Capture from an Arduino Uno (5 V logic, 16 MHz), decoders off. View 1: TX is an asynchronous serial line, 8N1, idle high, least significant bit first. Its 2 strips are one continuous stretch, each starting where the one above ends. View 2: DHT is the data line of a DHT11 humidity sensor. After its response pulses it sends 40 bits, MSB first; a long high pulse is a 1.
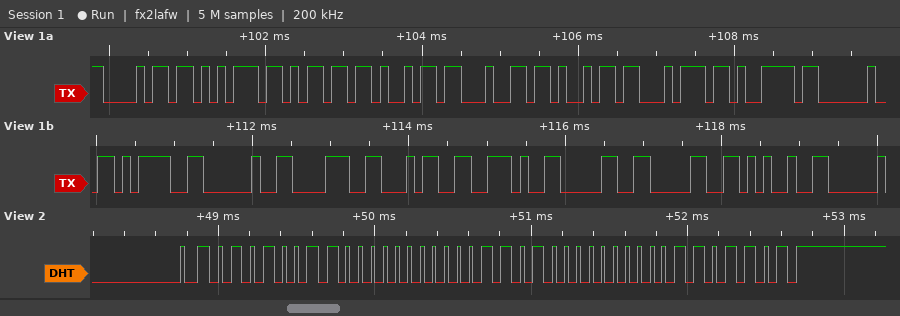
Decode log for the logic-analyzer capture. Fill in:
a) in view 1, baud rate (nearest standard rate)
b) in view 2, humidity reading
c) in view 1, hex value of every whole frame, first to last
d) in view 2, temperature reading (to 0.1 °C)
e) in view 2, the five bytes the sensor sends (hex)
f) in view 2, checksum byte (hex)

9600 baud
83 %
68 75 6D 69 64 69 74 79 20 3D 20 38 34 2E 30 30 25
26.0 °C
53 00 1A 00 6D
0x6D
